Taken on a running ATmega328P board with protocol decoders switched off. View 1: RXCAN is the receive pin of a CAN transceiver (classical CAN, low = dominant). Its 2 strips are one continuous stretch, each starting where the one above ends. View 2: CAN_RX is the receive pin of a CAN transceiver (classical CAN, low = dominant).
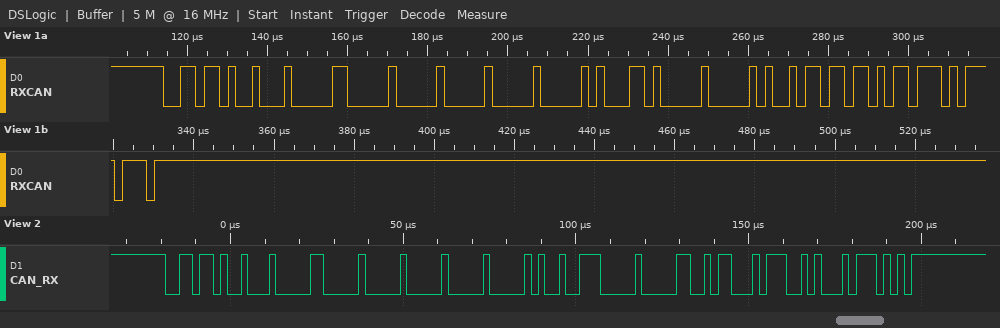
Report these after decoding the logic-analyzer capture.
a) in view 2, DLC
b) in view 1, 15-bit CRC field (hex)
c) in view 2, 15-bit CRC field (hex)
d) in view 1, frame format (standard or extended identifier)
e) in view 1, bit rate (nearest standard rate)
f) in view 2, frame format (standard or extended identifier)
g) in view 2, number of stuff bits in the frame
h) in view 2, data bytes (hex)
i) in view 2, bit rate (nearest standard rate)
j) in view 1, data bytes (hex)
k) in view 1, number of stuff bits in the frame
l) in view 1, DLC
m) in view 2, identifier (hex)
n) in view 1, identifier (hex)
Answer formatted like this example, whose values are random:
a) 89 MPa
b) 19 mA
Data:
a) 8
b) 0x6EBB
c) 0x28BA
d) standard
e) 500 kbit/s
f) standard
g) 8
h) 20 00 00 04 9C 00 96 2E
i) 500 kbit/s
j) 20 00 00 04 68 00 96 DA
k) 8
l) 8
m) 0x369
n) 0x369
